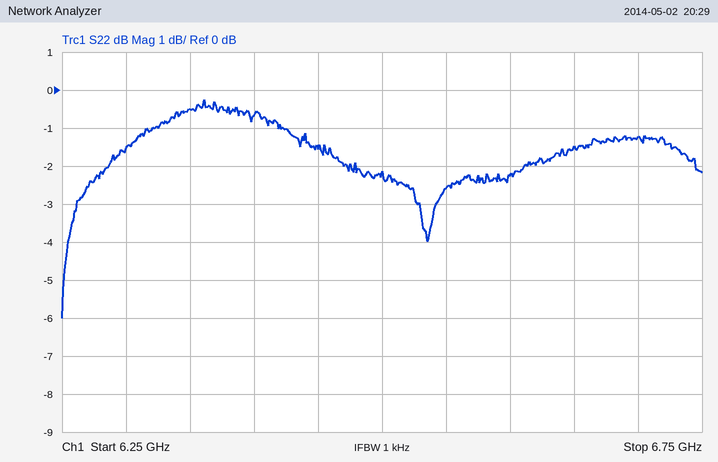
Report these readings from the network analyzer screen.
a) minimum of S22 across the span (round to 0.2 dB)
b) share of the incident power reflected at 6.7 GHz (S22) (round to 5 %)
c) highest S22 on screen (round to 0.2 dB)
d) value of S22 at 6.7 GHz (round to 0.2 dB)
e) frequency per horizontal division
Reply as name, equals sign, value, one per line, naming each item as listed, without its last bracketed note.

minimum of S22 across the span = -6.0 dB
share of the incident power reflected at 6.7 GHz (S22) = 75 %
highest S22 on screen = -0.2 dB
value of S22 at 6.7 GHz = -1.2 dB
frequency per horizontal division = 50 MHz
